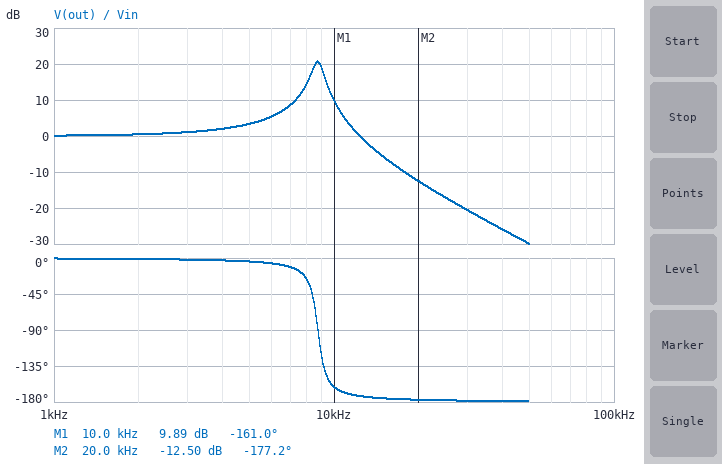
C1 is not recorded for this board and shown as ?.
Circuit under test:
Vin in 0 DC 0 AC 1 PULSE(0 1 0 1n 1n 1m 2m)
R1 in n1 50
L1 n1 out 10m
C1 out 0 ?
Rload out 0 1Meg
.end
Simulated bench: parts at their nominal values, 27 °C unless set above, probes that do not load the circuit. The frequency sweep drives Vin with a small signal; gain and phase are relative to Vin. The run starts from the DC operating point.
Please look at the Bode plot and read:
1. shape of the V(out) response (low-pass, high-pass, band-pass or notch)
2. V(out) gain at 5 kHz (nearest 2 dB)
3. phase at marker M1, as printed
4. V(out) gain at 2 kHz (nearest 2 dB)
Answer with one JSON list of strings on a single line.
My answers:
["low-pass", "4 dB", "-161.0 deg", "0 dB"]
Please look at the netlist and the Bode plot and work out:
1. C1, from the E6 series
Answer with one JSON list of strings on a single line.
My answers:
["33 nF"]
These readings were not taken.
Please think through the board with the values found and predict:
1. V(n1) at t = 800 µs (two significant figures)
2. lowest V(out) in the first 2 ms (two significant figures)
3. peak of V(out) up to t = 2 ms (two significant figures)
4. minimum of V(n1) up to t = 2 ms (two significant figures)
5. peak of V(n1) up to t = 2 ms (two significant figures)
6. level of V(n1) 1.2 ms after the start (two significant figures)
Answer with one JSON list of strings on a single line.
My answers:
["1.0 V", "-870 mV", "1.9 V", "-74 mV", "1.1 V", "-55 mV"]
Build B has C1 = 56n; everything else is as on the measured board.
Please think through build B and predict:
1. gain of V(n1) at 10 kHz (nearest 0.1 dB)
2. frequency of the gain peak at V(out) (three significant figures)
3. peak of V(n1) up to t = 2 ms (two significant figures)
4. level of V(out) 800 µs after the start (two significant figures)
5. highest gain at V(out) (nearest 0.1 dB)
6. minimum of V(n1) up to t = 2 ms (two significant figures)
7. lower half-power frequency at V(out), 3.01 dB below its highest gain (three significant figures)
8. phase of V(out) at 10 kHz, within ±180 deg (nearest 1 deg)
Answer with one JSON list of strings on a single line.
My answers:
["-0.1 dB", "6.70 kHz", "1.1 V", "1.1 V", "18.5 dB", "-92 mV", "6.29 kHz", "-172 deg"]
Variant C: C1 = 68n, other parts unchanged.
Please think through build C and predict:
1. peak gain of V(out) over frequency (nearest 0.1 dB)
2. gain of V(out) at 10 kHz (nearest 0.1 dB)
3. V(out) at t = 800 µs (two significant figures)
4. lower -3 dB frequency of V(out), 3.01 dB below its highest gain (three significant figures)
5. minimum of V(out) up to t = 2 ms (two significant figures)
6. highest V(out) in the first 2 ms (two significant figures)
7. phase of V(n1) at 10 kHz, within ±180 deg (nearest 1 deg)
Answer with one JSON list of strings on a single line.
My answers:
["17.7 dB", "-4.6 dB", "910 mV", "5.66 kHz", "-760 mV", "1.8 V", "7 deg"]
